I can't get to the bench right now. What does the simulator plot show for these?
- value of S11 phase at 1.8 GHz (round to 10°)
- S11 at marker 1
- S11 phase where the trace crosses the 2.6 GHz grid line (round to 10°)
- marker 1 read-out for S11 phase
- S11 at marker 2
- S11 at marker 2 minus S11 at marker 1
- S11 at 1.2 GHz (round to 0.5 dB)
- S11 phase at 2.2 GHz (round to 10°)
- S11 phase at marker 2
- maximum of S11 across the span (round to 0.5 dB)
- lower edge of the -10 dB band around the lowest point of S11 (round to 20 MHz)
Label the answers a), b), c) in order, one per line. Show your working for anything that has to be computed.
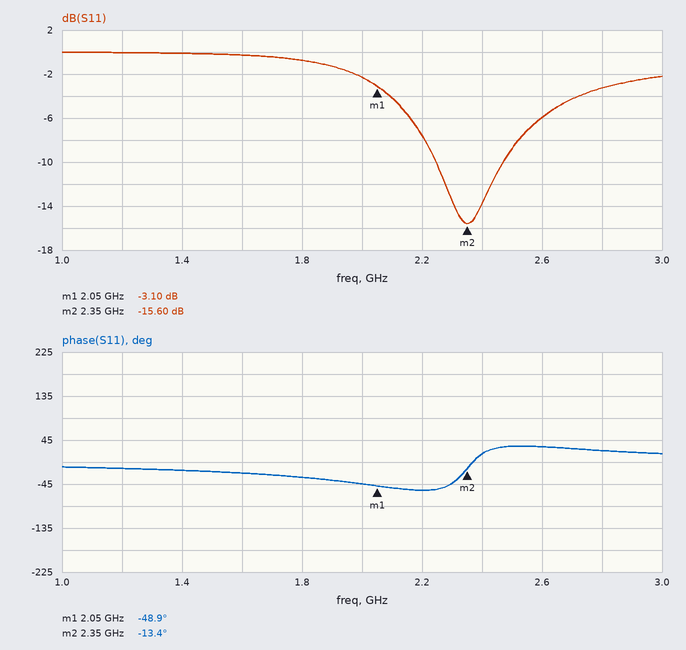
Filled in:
a) -30°
b) -3.10 dB
c) 30°
d) -48.9°
e) -15.60 dB
f) -15.6 − (-3.1) = -12.50 dB
g) 0.0 dB
h) -60°
i) -13.4°
j) 0.0 dB
k) 2.24 GHz
